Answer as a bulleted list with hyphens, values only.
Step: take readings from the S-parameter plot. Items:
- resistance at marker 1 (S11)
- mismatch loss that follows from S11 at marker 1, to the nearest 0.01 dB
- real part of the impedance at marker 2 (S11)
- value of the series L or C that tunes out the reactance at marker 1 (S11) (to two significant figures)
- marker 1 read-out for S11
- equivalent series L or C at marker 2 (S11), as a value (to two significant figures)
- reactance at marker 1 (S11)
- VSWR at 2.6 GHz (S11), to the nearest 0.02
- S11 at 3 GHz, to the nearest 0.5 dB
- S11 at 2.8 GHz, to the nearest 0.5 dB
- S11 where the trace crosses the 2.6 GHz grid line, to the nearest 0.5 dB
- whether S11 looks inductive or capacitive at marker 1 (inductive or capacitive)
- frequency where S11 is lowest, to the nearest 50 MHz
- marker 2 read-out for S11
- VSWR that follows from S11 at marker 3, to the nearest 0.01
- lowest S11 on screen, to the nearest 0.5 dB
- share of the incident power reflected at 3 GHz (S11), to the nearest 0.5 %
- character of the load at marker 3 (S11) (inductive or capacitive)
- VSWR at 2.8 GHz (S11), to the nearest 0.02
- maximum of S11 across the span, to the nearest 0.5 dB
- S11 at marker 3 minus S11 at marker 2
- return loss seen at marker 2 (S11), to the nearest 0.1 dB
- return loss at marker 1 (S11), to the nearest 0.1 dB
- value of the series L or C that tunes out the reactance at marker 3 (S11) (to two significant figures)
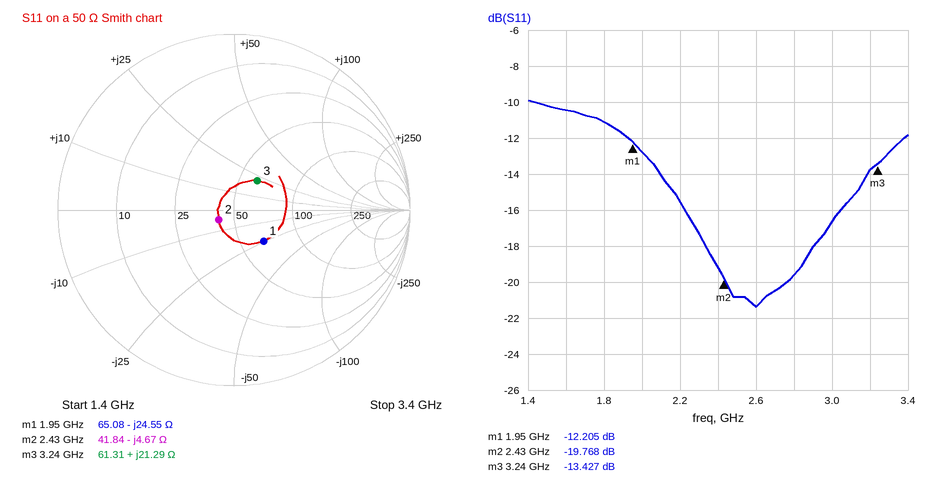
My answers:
- 65.08 Ω
- 0.27 dB
- 41.84 Ω
- 2.0 nH
- -12.205 dB
- 14 pF
- -24.55 Ω
- 1.18
- -16.5 dB
- -19.5 dB
- -21.5 dB
- capacitive
- 2.60 GHz
- -19.768 dB
- 1.54
- -21.5 dB
- 2.0 %
- inductive
- 1.24
- -10.0 dB
- 6.341 dB
- 19.8 dB
- 12.2 dB
- 2.3 pF
